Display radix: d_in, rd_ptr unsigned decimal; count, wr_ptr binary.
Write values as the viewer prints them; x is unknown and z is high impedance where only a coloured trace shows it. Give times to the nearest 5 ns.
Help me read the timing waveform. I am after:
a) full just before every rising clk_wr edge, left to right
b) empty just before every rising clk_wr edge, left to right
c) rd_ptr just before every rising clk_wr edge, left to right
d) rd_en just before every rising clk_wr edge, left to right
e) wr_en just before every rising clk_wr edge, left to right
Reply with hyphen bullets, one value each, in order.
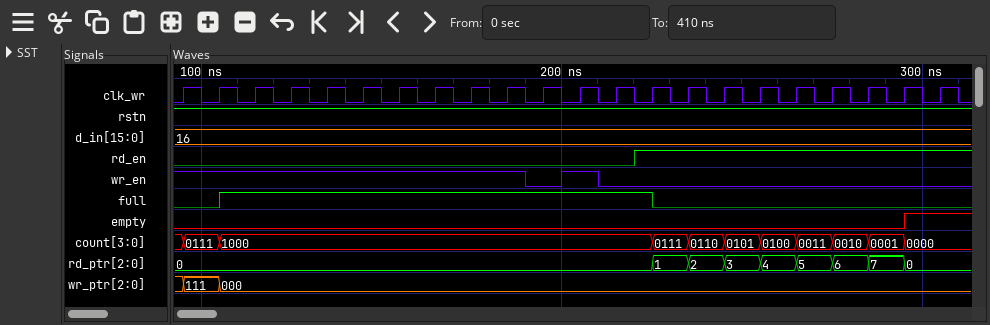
- 0 0 1 1 1 1 1 1 1 1 1 1 1 1 0 0 0 0 0 0 0 0
- 0 0 0 0 0 0 0 0 0 0 0 0 0 0 0 0 0 0 0 0 0 1
- 0, 0, 0, 0, 0, 0, 0, 0, 0, 0, 0, 0, 0, 0, 1, 2, 3, 4, 5, 6, 7, 0
- 0 0 0 0 0 0 0 0 0 0 0 0 0 1 1 1 1 1 1 1 1 1
- 1 1 1 1 1 1 1 1 1 1 0 1 0 0 0 0 0 0 0 0 0 0
